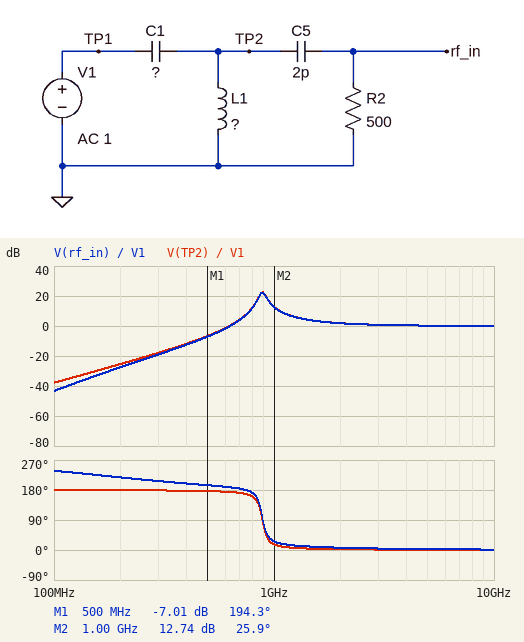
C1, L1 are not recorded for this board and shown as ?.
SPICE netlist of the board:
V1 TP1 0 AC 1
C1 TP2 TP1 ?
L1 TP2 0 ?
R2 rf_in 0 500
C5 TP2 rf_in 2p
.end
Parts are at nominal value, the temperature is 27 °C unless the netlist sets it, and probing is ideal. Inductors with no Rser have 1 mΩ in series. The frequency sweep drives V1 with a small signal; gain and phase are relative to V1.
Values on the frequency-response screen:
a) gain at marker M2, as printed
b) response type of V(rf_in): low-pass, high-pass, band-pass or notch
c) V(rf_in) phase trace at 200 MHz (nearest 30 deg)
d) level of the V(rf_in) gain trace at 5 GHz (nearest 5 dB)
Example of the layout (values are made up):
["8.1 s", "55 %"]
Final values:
["12.74 dB", "high-pass", "210 deg", "0 dB"]
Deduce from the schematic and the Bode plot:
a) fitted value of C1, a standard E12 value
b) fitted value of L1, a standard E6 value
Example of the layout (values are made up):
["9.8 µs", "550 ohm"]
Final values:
["4.7 pF", "6.8 nH"]
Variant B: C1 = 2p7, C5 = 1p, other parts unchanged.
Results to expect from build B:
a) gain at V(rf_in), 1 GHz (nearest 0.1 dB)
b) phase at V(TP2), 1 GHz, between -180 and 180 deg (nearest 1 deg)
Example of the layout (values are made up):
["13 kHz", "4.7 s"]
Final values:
["8.4 dB", "163 deg"]
